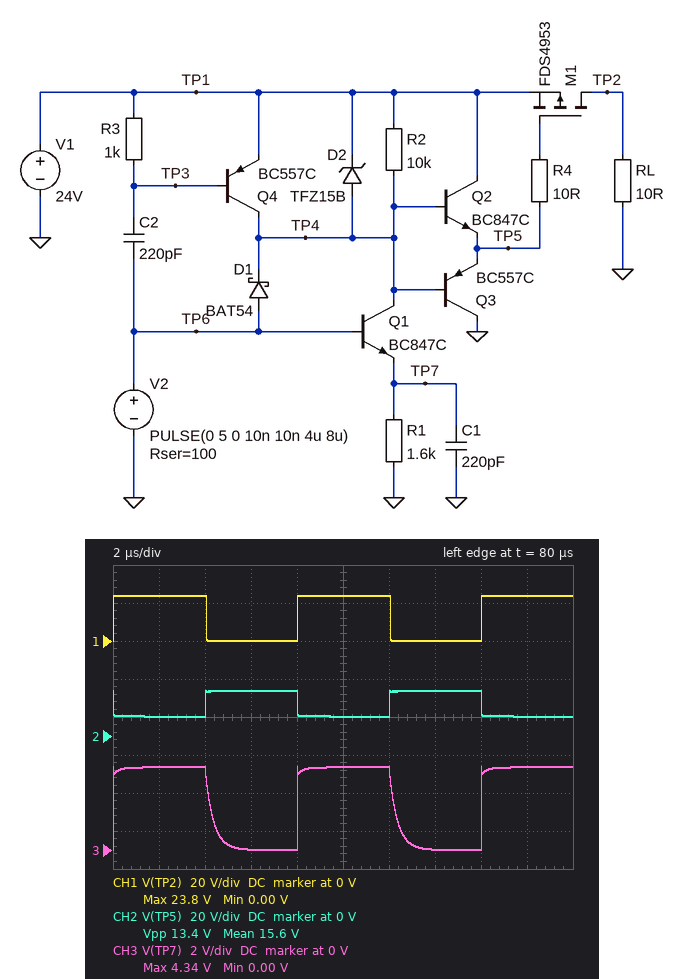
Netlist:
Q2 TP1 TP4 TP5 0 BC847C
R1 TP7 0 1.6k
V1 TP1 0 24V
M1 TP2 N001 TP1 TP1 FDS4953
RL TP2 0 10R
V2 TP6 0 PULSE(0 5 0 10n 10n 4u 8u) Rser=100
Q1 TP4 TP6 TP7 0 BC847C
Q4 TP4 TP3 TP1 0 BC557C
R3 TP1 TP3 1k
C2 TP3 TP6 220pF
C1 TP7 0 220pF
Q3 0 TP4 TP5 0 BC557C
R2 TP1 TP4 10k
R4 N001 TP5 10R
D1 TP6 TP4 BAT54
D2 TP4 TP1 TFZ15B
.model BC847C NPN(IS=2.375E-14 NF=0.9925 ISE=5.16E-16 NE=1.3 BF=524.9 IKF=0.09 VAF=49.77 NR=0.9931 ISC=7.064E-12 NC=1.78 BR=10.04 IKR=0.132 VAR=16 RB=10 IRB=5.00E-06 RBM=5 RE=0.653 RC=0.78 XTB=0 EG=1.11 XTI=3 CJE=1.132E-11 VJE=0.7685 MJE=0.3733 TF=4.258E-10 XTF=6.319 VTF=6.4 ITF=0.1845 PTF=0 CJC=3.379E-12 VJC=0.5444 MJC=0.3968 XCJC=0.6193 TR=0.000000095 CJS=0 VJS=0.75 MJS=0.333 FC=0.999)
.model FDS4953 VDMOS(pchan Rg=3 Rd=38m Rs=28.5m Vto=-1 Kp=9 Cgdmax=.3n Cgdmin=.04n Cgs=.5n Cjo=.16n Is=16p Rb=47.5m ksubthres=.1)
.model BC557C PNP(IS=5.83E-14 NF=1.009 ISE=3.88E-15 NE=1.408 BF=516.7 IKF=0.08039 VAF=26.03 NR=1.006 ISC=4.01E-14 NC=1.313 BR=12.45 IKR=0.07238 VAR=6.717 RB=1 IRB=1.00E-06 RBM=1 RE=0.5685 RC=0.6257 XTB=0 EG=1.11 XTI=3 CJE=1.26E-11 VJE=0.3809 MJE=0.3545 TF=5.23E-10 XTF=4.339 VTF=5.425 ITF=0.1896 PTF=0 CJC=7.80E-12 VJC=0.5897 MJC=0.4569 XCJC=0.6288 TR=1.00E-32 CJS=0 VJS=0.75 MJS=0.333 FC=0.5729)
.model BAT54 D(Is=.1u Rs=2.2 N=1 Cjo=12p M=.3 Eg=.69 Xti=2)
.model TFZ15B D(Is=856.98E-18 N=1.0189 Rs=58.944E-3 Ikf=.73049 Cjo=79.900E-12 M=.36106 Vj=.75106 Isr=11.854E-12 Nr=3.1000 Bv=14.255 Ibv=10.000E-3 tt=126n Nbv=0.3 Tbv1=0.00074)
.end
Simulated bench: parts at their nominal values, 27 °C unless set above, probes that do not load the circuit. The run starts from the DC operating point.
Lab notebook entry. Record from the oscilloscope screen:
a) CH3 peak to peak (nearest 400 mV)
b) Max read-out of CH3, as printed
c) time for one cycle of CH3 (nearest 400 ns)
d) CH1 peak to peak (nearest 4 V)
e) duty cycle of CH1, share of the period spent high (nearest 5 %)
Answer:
4.4 V
4.34 V
8.0 µs
24 V
50 %
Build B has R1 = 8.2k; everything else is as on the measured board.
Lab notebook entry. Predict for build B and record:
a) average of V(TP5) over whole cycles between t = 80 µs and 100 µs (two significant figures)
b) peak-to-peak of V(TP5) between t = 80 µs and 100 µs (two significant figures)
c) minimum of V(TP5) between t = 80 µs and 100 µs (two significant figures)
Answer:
20 V
11 V
12 V
